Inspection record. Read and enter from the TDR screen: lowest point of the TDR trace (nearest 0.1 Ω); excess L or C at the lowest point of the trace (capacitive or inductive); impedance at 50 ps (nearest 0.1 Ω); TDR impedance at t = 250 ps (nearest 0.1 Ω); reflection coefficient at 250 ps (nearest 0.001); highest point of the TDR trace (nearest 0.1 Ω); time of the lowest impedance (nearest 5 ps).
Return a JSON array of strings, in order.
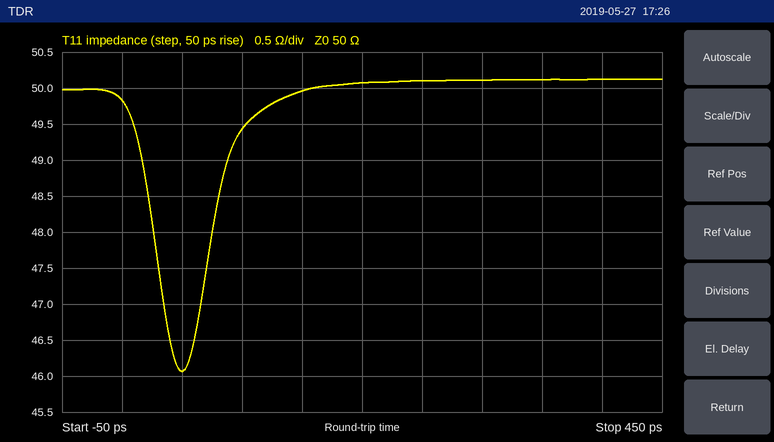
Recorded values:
["46.1 Ω", "capacitive", "46.1 Ω", "50.1 Ω", "+0.001", "50.1 Ω", "50 ps"]
